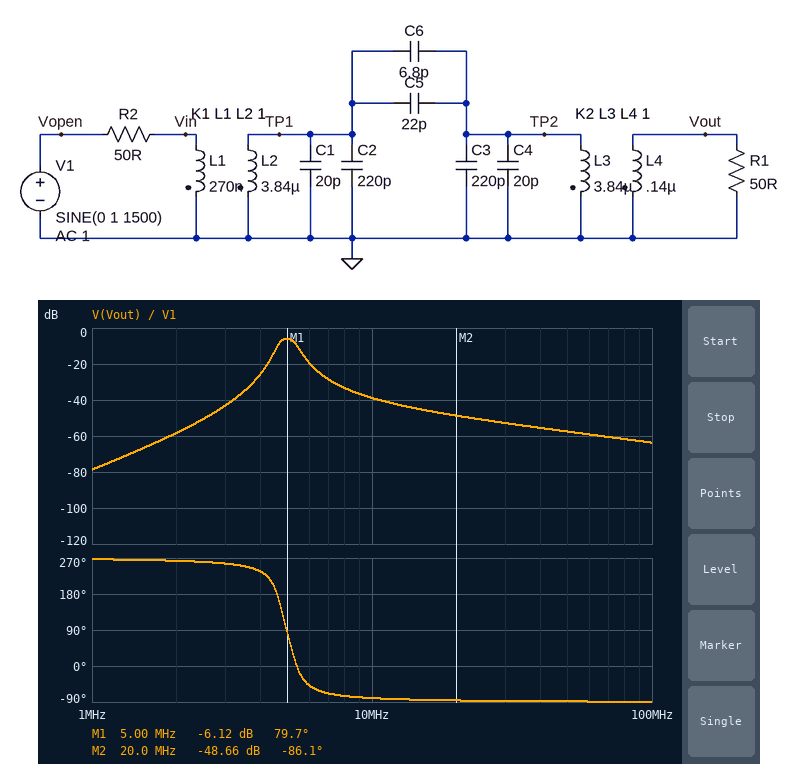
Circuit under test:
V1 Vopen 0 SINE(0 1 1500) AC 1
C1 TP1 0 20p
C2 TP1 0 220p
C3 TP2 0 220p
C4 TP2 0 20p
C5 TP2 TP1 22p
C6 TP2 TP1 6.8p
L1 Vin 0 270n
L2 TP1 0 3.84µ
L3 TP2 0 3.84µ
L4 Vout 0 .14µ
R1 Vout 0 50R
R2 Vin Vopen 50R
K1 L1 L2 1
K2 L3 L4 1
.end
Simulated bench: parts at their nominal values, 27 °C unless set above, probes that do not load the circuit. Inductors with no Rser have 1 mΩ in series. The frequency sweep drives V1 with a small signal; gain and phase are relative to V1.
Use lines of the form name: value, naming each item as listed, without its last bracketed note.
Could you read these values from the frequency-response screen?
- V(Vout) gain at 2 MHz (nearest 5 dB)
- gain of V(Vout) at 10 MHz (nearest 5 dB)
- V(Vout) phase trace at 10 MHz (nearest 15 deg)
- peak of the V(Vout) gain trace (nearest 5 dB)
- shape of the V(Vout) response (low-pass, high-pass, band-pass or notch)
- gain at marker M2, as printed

V(Vout) gain at 2 MHz: -60 dB
gain of V(Vout) at 10 MHz: -40 dB
V(Vout) phase trace at 10 MHz: -75 deg
peak of the V(Vout) gain trace: -5 dB
shape of the V(Vout) response: band-pass
gain at marker M2, as printed: -48.66 dB
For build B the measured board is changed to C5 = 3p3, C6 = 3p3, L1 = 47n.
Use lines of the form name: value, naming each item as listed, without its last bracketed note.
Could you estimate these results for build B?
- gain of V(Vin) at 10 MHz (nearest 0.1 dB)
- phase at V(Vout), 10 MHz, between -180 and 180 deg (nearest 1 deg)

gain of V(Vin) at 10 MHz: -33.3 dB
phase at V(Vout), 10 MHz, between -180 and 180 deg: -85 deg
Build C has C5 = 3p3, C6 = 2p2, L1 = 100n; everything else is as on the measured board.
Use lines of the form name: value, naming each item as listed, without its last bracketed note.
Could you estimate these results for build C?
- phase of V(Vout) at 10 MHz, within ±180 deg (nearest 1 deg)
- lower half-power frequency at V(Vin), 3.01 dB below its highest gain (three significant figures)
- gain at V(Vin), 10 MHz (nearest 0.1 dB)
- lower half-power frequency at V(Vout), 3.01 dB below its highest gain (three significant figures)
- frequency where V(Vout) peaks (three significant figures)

phase of V(Vout) at 10 MHz, within ±180 deg: -84 deg
lower half-power frequency at V(Vin), 3.01 dB below its highest gain: 4.99 MHz
gain at V(Vin), 10 MHz: -26.7 dB
lower half-power frequency at V(Vout), 3.01 dB below its highest gain: 5.05 MHz
frequency where V(Vout) peaks: 5.19 MHz
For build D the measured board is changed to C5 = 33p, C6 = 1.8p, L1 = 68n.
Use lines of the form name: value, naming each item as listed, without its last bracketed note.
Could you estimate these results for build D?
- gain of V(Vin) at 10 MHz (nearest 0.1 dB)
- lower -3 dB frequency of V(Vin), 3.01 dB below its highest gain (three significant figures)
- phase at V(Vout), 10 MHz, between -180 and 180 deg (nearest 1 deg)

gain of V(Vin) at 10 MHz: -31.1 dB
lower -3 dB frequency of V(Vin), 3.01 dB below its highest gain: 4.45 MHz
phase at V(Vout), 10 MHz, between -180 and 180 deg: -85 deg
